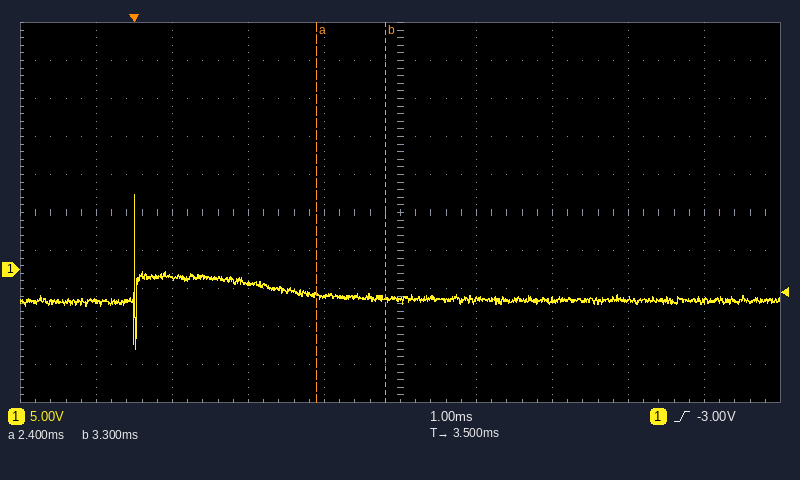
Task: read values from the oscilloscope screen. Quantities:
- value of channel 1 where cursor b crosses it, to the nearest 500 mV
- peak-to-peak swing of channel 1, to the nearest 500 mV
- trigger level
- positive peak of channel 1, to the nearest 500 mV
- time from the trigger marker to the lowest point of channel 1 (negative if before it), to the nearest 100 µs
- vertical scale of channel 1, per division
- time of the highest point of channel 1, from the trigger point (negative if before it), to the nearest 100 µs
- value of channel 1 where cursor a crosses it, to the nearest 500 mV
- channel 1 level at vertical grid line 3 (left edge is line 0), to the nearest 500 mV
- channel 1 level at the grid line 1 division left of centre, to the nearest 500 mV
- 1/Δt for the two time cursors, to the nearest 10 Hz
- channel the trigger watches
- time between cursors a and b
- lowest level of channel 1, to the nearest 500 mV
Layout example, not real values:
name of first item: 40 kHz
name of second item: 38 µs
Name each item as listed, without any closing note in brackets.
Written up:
value of channel 1 where cursor b crosses it, to the nearest 500 mV: -4.0 V
peak-to-peak swing of channel 1, to the nearest 500 mV: 20.5 V
trigger level: -3.00 V
positive peak of channel 1, to the nearest 500 mV: 10.0 V
time from the trigger marker to the lowest point of channel 1 (negative if before it), to the nearest 100 µs: 0.0 ms
vertical scale of channel 1, per division: 5 V
time of the highest point of channel 1, from the trigger point (negative if before it), to the nearest 100 µs: 0.0 ms
value of channel 1 where cursor a crosses it, to the nearest 500 mV: -3.5 V
channel 1 level at vertical grid line 3 (left edge is line 0), to the nearest 500 mV: -2.0 V
channel 1 level at the grid line 1 division left of centre, to the nearest 500 mV: -3.5 V
1/Δt for the two time cursors, to the nearest 10 Hz: 1.11 kHz
channel the trigger watches: channel 1
time between cursors a and b: 900 µs
lowest level of channel 1, to the nearest 500 mV: -10.5 V
